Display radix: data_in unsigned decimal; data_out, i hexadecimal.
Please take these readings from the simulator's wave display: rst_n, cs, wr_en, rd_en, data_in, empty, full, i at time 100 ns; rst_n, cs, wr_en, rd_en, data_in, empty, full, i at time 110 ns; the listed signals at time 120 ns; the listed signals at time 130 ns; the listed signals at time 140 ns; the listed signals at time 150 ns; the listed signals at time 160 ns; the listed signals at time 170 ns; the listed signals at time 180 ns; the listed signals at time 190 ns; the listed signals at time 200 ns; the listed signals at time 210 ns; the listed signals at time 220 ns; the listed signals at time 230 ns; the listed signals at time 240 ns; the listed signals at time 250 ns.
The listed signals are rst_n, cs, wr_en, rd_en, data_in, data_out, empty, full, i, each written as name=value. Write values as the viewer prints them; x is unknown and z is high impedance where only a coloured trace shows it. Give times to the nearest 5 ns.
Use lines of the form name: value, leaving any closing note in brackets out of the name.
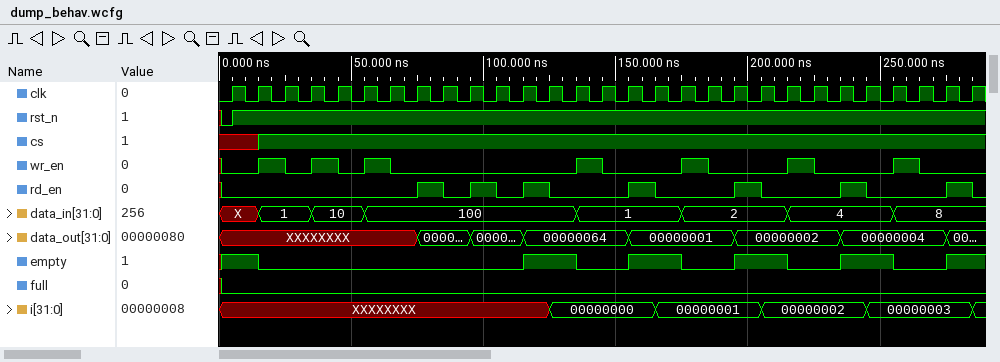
rst_n, cs, wr_en, rd_en, data_in, empty, full, i at time 100 ns: rst_n=1, cs=1, wr_en=0, rd_en=1, data_in=100, empty=0, full=0, i=XXXXXXXX
rst_n, cs, wr_en, rd_en, data_in, empty, full, i at time 110 ns: rst_n=1, cs=1, wr_en=0, rd_en=0, data_in=100, empty=0, full=0, i=XXXXXXXX
the listed signals at time 120 ns: rst_n=1, cs=1, wr_en=0, rd_en=1, data_in=100, data_out=00000064, empty=1, full=0, i=XXXXXXXX
the listed signals at time 130 ns: rst_n=1, cs=1, wr_en=0, rd_en=0, data_in=100, data_out=00000064, empty=1, full=0, i=00000000
the listed signals at time 140 ns: rst_n=1, cs=1, wr_en=1, rd_en=0, data_in=1, data_out=00000064, empty=0, full=0, i=00000000
the listed signals at time 150 ns: rst_n=1, cs=1, wr_en=0, rd_en=0, data_in=1, data_out=00000064, empty=0, full=0, i=00000000
the listed signals at time 160 ns: rst_n=1, cs=1, wr_en=0, rd_en=1, data_in=1, data_out=00000001, empty=1, full=0, i=00000000
the listed signals at time 170 ns: rst_n=1, cs=1, wr_en=0, rd_en=0, data_in=1, data_out=00000001, empty=1, full=0, i=00000001
the listed signals at time 180 ns: rst_n=1, cs=1, wr_en=1, rd_en=0, data_in=2, data_out=00000001, empty=0, full=0, i=00000001
the listed signals at time 190 ns: rst_n=1, cs=1, wr_en=0, rd_en=0, data_in=2, data_out=00000001, empty=0, full=0, i=00000001
the listed signals at time 200 ns: rst_n=1, cs=1, wr_en=0, rd_en=1, data_in=2, data_out=00000002, empty=1, full=0, i=00000001
the listed signals at time 210 ns: rst_n=1, cs=1, wr_en=0, rd_en=0, data_in=2, data_out=00000002, empty=1, full=0, i=00000002
the listed signals at time 220 ns: rst_n=1, cs=1, wr_en=1, rd_en=0, data_in=4, data_out=00000002, empty=0, full=0, i=00000002
the listed signals at time 230 ns: rst_n=1, cs=1, wr_en=0, rd_en=0, data_in=4, data_out=00000002, empty=0, full=0, i=00000002
the listed signals at time 240 ns: rst_n=1, cs=1, wr_en=0, rd_en=1, data_in=4, data_out=00000004, empty=1, full=0, i=00000002
the listed signals at time 250 ns: rst_n=1, cs=1, wr_en=0, rd_en=0, data_in=4, data_out=00000004, empty=1, full=0, i=00000003
